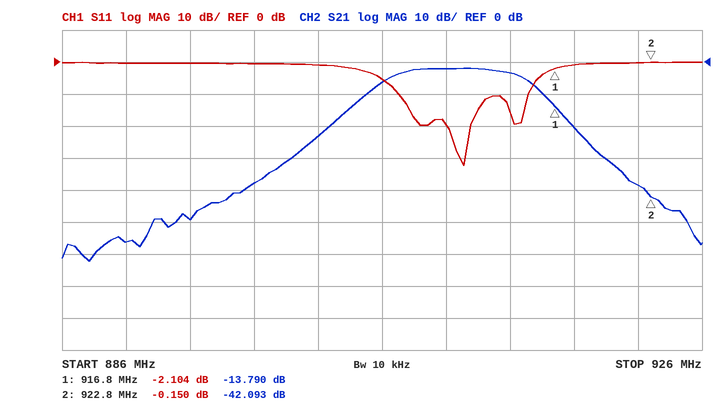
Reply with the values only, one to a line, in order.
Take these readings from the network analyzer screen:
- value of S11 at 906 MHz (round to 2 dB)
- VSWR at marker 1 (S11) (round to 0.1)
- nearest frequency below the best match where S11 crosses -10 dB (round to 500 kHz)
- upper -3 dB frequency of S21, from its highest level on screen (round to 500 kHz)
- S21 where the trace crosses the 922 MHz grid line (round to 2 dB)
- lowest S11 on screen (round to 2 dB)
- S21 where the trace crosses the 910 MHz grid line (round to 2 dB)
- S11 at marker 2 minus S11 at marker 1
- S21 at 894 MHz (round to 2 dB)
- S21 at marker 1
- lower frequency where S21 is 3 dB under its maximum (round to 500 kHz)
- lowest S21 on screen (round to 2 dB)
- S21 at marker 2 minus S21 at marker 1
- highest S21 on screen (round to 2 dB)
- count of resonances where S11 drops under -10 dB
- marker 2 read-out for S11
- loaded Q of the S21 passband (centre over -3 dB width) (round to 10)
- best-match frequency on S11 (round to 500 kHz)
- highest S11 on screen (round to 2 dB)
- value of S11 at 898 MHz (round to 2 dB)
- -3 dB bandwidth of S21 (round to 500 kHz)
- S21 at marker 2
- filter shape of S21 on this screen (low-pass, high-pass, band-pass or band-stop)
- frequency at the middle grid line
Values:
-6 dB
8.3
907.0 MHz
915.0 MHz
-38 dB
-32 dB
-2 dB
1.954 dB
-50 dB
-13.790 dB
906.5 MHz
-62 dB
-28.303 dB
-2 dB
2
-0.150 dB
110
911.0 MHz
0 dB
0 dB
8.5 MHz
-42.093 dB
band-pass
906 MHz
